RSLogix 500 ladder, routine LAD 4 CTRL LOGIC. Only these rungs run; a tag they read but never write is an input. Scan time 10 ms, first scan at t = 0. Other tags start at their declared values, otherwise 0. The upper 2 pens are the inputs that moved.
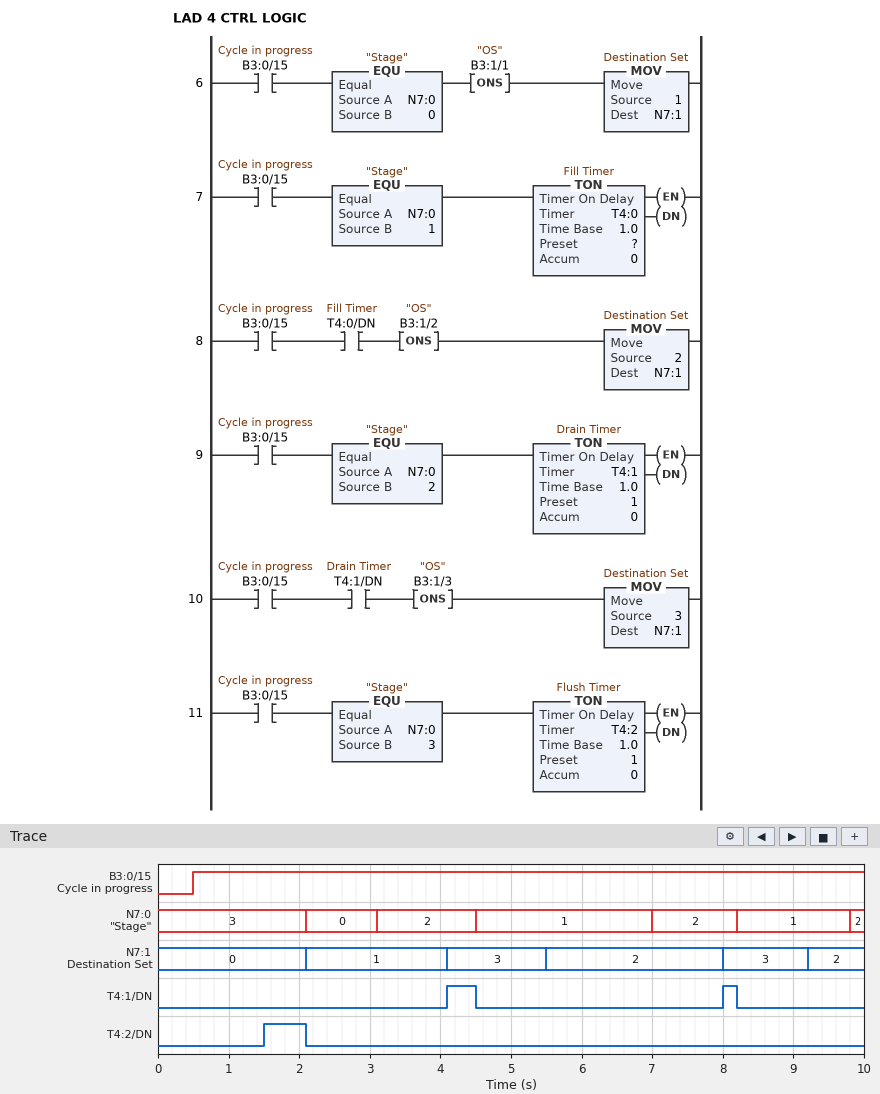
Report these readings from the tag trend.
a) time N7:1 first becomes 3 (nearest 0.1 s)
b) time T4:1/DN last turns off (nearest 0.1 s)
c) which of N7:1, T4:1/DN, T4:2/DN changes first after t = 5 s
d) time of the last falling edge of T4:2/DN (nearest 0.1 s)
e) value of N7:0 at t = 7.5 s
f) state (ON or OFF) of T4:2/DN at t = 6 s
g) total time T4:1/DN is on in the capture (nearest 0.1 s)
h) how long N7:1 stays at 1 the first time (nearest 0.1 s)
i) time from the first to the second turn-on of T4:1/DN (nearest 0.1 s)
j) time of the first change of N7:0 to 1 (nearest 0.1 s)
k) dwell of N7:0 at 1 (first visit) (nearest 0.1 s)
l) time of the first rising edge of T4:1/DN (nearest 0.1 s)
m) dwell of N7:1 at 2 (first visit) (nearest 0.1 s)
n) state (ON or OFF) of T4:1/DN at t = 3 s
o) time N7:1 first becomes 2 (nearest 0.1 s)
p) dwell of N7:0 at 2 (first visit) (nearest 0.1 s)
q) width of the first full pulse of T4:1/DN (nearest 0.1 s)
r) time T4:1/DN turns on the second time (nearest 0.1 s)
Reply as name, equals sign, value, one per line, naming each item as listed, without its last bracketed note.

time N7:1 first becomes 3 = 4.1 s
time T4:1/DN last turns off = 8.2 s
which of N7:1, T4:1/DN, T4:2/DN changes first after t = 5 s = N7:1
time of the last falling edge of T4:2/DN = 2.1 s
value of N7:0 at t = 7.5 s = 2
state (ON or OFF) of T4:2/DN at t = 6 s = OFF
total time T4:1/DN is on in the capture = 0.6 s
how long N7:1 stays at 1 the first time = 2.0 s
time from the first to the second turn-on of T4:1/DN = 3.9 s
time of the first change of N7:0 to 1 = 4.5 s
dwell of N7:0 at 1 (first visit) = 2.5 s
time of the first rising edge of T4:1/DN = 4.1 s
dwell of N7:1 at 2 (first visit) = 2.5 s
state (ON or OFF) of T4:1/DN at t = 3 s = OFF
time N7:1 first becomes 2 = 5.5 s
dwell of N7:0 at 2 (first visit) = 1.4 s
width of the first full pulse of T4:1/DN = 0.4 s
time T4:1/DN turns on the second time = 8.0 s
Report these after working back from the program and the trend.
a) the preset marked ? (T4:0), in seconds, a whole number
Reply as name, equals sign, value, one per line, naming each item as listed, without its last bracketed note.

the preset marked ? (T4:0), in seconds, a whole number = 1 s
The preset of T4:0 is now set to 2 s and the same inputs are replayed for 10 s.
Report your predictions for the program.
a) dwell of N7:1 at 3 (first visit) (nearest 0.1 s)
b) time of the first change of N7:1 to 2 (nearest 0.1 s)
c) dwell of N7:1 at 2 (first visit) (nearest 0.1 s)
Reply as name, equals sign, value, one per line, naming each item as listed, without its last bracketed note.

dwell of N7:1 at 3 (first visit) = 2.4 s
time of the first change of N7:1 to 2 = 6.5 s
dwell of N7:1 at 2 (first visit) = 1.5 s
